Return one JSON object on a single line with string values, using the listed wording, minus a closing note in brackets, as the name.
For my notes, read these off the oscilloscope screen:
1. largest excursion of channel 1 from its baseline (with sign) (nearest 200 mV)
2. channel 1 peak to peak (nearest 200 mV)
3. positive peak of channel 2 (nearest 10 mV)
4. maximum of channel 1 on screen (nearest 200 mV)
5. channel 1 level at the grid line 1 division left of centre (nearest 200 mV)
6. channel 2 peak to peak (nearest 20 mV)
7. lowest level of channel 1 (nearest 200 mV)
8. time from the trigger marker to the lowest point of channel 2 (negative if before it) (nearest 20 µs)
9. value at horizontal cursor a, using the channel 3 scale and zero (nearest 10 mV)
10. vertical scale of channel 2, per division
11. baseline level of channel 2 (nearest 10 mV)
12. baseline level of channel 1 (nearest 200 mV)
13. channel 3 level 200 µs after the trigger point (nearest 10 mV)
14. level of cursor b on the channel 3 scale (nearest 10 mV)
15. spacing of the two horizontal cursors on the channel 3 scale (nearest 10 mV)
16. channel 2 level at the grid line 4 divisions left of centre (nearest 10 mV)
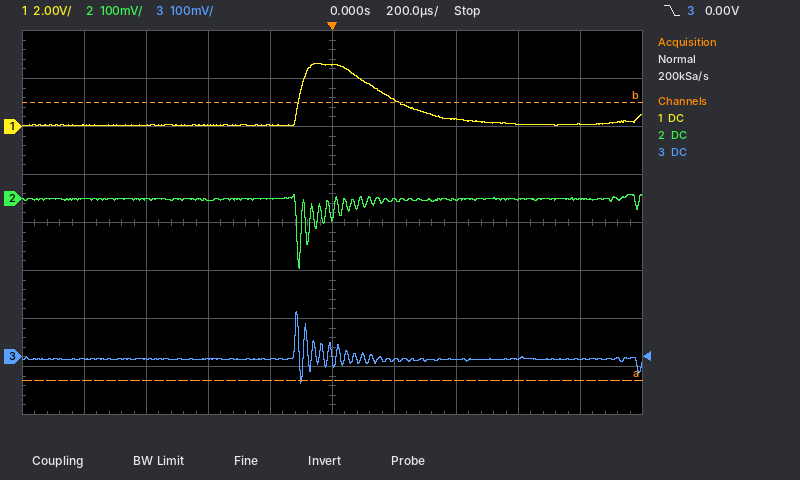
{"largest excursion of channel 1 from its baseline (with sign)": "+2.6 V", "channel 1 peak to peak": "2.6 V", "positive peak of channel 2": "10 mV", "maximum of channel 1 on screen": "2.6 V", "channel 1 level at the grid line 1 division left of centre": "0.0 V", "channel 2 peak to peak": "160 mV", "lowest level of channel 1": "0.0 V", "time from the trigger marker to the lowest point of channel 2 (negative if before it)": "-100 µs", "value at horizontal cursor a, using the channel 3 scale and zero": "-50 mV", "vertical scale of channel 2, per division": "100 mV", "baseline level of channel 2": "0 mV", "baseline level of channel 1": "0.0 V", "channel 3 level 200 µs after the trigger point": "-10 mV", "level of cursor b on the channel 3 scale": "530 mV", "spacing of the two horizontal cursors on the channel 3 scale": "580 mV", "channel 2 level at the grid line 4 divisions left of centre": "0 mV"}
